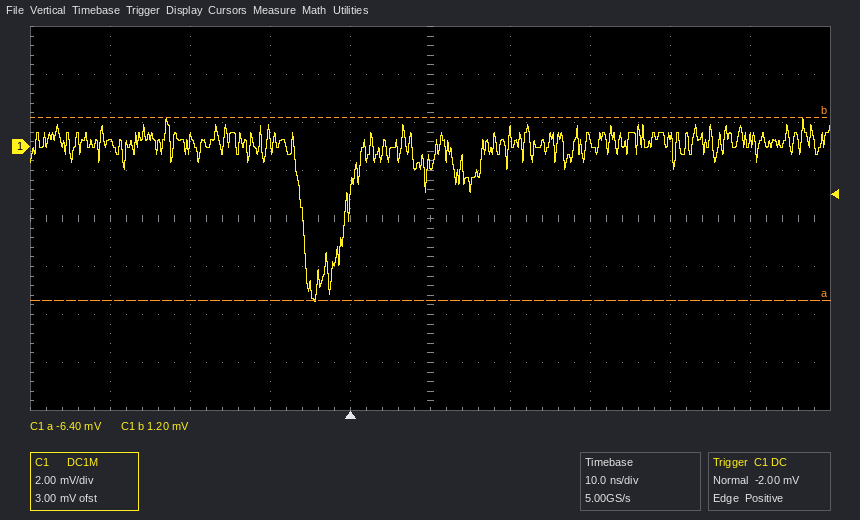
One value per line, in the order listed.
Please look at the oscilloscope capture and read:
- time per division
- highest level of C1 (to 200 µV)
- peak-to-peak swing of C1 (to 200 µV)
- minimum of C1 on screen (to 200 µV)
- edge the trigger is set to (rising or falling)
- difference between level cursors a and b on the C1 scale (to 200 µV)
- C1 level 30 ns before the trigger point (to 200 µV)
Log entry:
10 ns
1.2 mV
7.6 mV
-6.4 mV
rising
7.6 mV
200 µV
